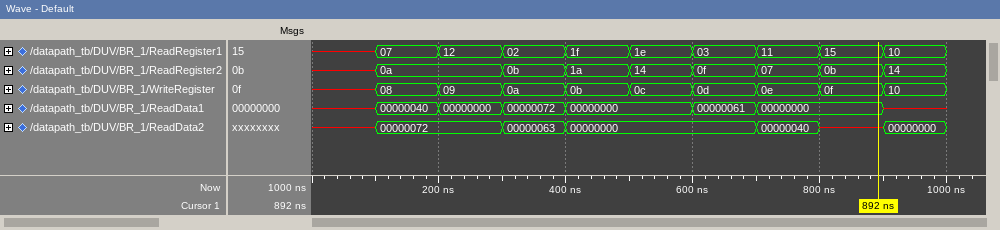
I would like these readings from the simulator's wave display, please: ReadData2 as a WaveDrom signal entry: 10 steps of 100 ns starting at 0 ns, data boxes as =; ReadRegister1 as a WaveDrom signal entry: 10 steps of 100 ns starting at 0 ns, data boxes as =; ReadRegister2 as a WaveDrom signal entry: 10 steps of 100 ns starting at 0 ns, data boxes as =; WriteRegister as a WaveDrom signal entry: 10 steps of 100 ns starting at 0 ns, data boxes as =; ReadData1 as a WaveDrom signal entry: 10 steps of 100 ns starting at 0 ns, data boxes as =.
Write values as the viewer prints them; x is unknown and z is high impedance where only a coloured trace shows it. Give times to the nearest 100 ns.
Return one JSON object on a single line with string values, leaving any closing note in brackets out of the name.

{"ReadData2 as a WaveDrom signal entry: 10 steps of 100 ns starting at 0 ns, data boxes as =": "{name: 'ReadData2', wave: 'x=.==..=x=', data: '00000072 00000063 00000000 00000040 00000000'}", "ReadRegister1 as a WaveDrom signal entry: 10 steps of 100 ns starting at 0 ns, data boxes as =": "{name: 'ReadRegister1', wave: 'x=========', data: '07 12 02 1f 1e 03 11 15 10'}", "ReadRegister2 as a WaveDrom signal entry: 10 steps of 100 ns starting at 0 ns, data boxes as =": "{name: 'ReadRegister2', wave: 'x=.=======', data: '0a 0b 1a 14 0f 07 0b 14'}", "WriteRegister as a WaveDrom signal entry: 10 steps of 100 ns starting at 0 ns, data boxes as =": "{name: 'WriteRegister', wave: 'x=========', data: '08 09 0a 0b 0c 0d 0e 0f 10'}", "ReadData1 as a WaveDrom signal entry: 10 steps of 100 ns starting at 0 ns, data boxes as =": "{name: 'ReadData1', wave: 'x====.==.x', data: '00000040 00000000 00000072 00000000 00000061 00000000'}"}
